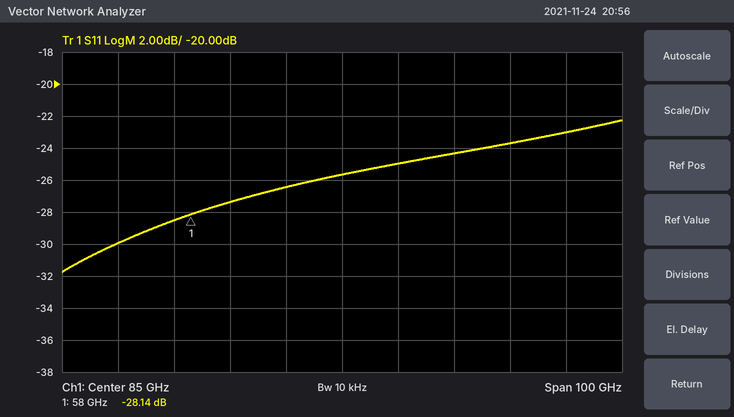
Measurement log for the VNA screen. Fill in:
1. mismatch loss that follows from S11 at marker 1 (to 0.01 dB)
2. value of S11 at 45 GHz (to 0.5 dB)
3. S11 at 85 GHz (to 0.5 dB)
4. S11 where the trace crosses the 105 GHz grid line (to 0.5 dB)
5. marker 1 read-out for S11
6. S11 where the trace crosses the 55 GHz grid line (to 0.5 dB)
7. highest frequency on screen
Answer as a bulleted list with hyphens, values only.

- 0.01 dB
- -30.0 dB
- -25.5 dB
- -24.5 dB
- -28.14 dB
- -28.5 dB
- 135 GHz
